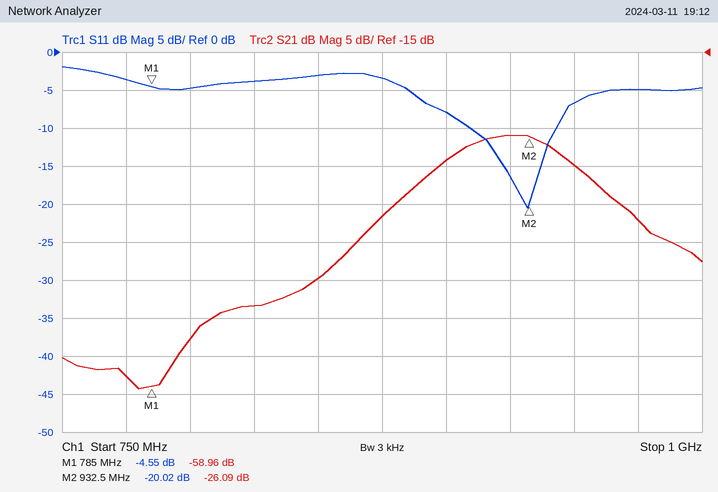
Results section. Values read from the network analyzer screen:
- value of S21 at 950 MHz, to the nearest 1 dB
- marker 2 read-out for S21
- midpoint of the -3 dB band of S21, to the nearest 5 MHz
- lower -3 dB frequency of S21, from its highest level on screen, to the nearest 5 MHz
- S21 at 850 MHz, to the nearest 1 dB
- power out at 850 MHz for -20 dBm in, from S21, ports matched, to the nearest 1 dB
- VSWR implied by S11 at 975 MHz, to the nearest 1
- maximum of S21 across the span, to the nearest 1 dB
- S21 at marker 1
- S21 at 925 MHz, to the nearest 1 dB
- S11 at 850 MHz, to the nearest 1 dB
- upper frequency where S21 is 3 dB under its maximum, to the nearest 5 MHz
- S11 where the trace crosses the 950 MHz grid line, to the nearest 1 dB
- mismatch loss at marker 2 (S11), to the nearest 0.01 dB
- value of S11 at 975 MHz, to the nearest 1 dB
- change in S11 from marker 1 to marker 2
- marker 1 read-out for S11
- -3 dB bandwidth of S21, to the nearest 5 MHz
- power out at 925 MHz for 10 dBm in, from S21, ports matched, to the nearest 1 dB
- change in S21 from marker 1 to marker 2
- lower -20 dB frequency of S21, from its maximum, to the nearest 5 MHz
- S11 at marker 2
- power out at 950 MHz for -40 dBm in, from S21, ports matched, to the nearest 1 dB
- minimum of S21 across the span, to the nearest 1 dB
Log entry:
-30 dB
-26.09 dB
925 MHz
900 MHz
-45 dB
-65 dBm
4
-26 dB
-58.96 dB
-26 dB
-3 dB
945 MHz
-7 dB
0.04 dB
-5 dB
-15.47 dB
-4.55 dB
45 MHz
-16 dBm
32.87 dB
845 MHz
-20.02 dB
-70 dBm
-59 dB
